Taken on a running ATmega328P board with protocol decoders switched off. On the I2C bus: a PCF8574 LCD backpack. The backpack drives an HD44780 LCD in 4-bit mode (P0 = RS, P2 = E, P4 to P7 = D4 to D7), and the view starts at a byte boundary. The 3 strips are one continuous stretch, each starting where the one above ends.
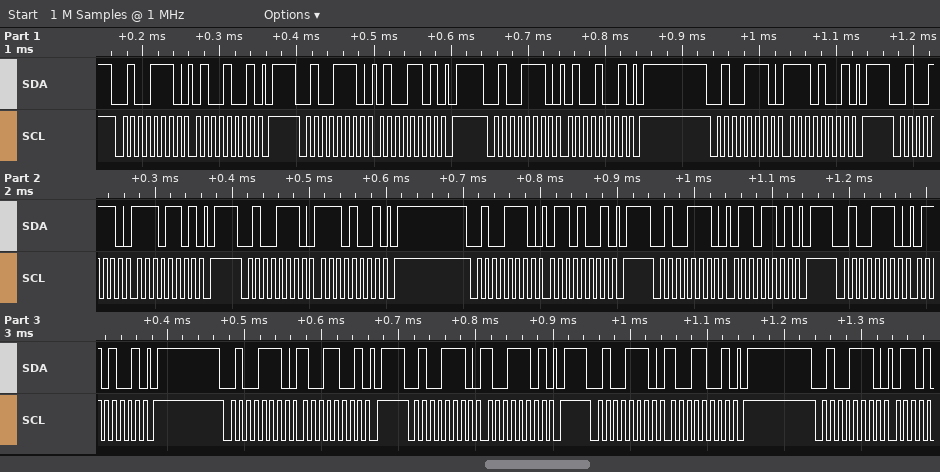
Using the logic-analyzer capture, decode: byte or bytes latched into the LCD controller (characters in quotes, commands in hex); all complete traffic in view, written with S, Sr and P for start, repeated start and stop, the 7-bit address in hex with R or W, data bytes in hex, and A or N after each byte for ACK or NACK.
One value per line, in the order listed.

'N' 'i'
S 27W A 49 A P S 27W A 4D A P S 27W A 49 A P S 27W A E9 A P S 27W A ED A P S 27W A E9 A P S 27W A 69 A P S 27W A 6D A P S 27W A 69 A P S 27W A 99 A P S 27W A 9D A P S 27W A 99 A P S 27W A
